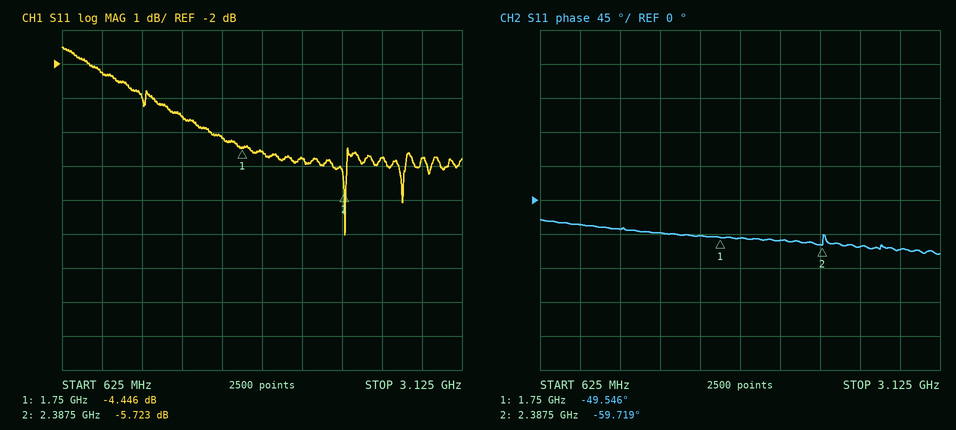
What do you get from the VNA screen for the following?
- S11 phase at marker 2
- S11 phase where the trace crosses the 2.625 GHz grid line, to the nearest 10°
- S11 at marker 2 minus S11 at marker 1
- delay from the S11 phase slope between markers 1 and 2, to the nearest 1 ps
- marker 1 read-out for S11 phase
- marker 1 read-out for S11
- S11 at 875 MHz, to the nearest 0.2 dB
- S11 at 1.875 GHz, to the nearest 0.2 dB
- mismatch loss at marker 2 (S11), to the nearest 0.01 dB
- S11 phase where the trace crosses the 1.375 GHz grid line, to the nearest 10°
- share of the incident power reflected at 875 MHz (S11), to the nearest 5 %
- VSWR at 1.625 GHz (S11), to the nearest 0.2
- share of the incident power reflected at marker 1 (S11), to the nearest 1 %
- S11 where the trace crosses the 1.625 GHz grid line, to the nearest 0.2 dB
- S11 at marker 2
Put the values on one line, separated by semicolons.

-59.719°; -60°; -1.277 dB; 44 ps; -49.546°; -4.446 dB; -2.2 dB; -4.6 dB; 1.35 dB; -40°; 60 %; 4.2; 36 %; -4.2 dB; -5.723 dB
